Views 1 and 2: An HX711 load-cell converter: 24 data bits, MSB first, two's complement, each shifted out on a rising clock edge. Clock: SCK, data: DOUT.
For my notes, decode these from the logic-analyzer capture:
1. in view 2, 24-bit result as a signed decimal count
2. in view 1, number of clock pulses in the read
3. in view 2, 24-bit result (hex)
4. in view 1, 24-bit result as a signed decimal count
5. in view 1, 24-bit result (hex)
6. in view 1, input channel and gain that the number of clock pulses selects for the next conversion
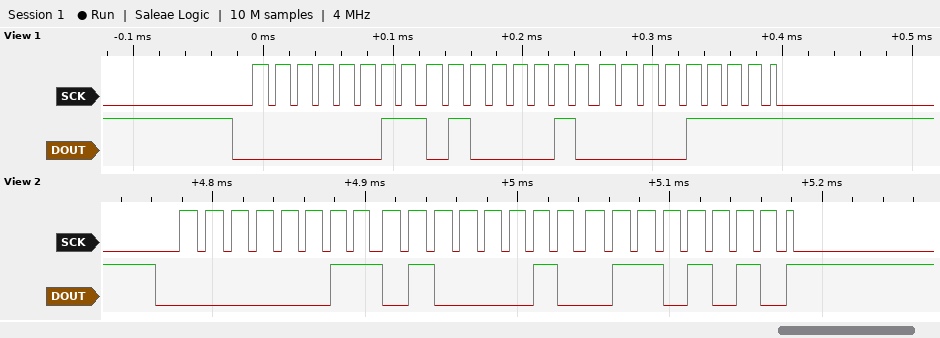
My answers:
213610
25
0x03426A
213519
0x03420F
channel A, gain 128
